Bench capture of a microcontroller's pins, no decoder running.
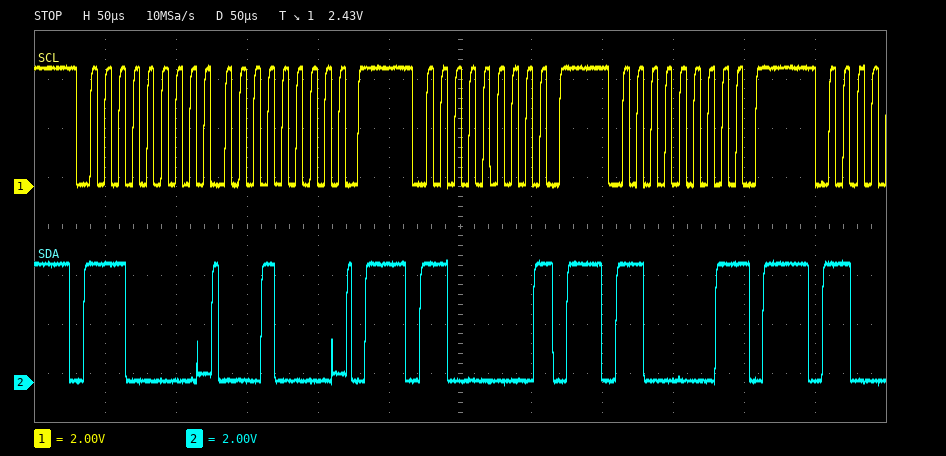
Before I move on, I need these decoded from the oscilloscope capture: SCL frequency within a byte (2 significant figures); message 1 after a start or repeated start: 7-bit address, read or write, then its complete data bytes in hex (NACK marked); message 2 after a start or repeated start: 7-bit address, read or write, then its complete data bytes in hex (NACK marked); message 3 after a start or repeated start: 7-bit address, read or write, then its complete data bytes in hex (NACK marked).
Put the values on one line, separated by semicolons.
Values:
100 kHz; 0x70 write: 10; 0x60 write NACK; 0x60 read NACK
